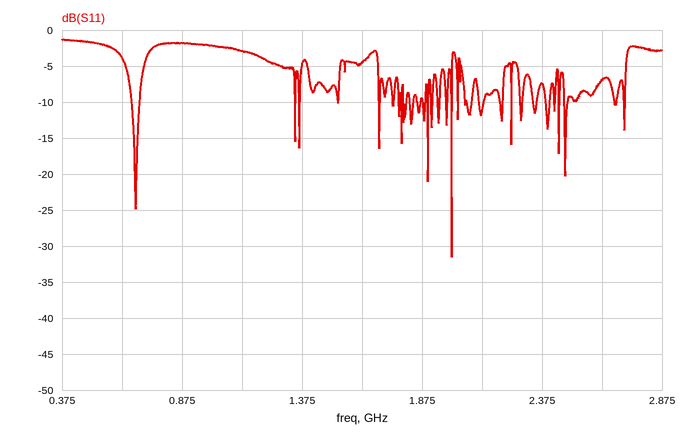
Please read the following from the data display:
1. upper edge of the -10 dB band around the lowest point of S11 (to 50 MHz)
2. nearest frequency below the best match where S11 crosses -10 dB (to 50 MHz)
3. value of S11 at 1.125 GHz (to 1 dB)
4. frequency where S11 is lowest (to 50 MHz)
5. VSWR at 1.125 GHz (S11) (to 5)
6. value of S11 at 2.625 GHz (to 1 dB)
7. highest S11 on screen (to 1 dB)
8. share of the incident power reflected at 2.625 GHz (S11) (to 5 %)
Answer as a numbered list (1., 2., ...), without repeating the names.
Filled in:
1. 2.00 GHz
2. 2.00 GHz
3. -3 dB
4. 2.00 GHz
5. 5
6. -7 dB
7. -1 dB
8. 20 %
